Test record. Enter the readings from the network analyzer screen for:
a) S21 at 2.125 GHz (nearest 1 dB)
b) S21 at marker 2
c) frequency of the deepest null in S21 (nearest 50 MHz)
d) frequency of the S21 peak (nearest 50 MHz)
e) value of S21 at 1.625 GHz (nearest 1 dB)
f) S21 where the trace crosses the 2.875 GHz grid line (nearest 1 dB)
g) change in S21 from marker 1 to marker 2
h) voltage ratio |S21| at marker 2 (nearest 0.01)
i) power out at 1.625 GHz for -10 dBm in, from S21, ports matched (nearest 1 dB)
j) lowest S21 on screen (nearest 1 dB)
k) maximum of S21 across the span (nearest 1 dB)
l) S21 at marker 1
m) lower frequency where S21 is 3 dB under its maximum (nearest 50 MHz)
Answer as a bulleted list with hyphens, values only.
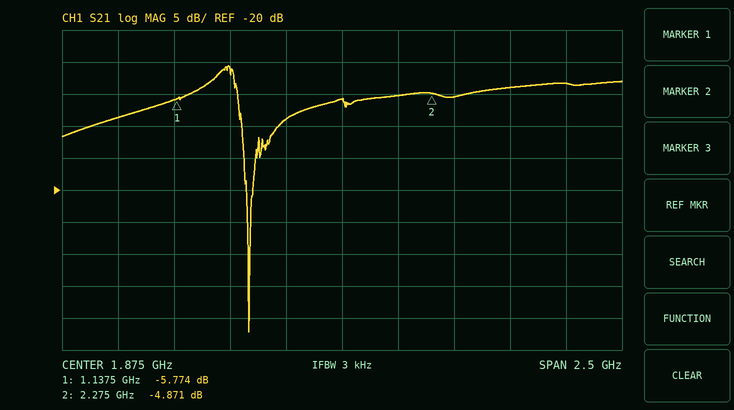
- -5 dB
- -4.871 dB
- 1.45 GHz
- 1.35 GHz
- -9 dB
- -3 dB
- 0.903 dB
- 0.57
- -19 dBm
- -42 dB
- -1 dB
- -5.774 dB
- 1.25 GHz
